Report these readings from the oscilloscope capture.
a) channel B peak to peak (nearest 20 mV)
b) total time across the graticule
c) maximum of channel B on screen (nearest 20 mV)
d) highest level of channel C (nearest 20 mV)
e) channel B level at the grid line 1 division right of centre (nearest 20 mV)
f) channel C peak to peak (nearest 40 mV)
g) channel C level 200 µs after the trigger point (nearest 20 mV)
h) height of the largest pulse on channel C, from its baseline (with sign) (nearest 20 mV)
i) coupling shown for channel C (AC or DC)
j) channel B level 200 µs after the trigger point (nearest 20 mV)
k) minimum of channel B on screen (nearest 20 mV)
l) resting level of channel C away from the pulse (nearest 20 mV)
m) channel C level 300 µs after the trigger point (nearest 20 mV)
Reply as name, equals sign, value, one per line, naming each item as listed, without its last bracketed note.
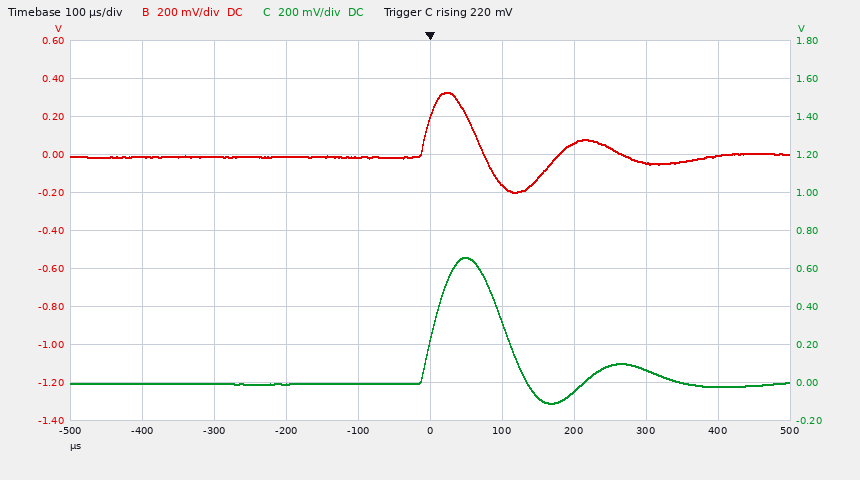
channel B peak to peak = 520 mV
total time across the graticule = 1 ms
maximum of channel B on screen = 320 mV
highest level of channel C = 660 mV
channel B level at the grid line 1 division right of centre = -160 mV
channel C peak to peak = 760 mV
channel C level 200 µs after the trigger point = -40 mV
height of the largest pulse on channel C, from its baseline (with sign) = +660 mV
coupling shown for channel C = DC
channel B level 200 µs after the trigger point = 60 mV
minimum of channel B on screen = -200 mV
resting level of channel C away from the pulse = 0 mV
channel C level 300 µs after the trigger point = 60 mV
